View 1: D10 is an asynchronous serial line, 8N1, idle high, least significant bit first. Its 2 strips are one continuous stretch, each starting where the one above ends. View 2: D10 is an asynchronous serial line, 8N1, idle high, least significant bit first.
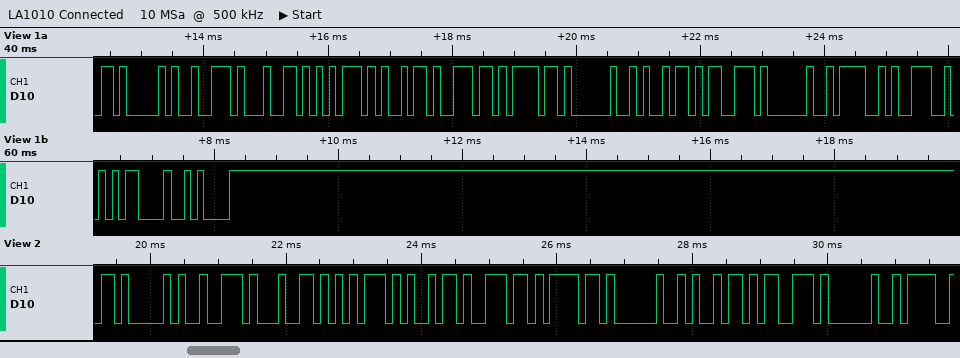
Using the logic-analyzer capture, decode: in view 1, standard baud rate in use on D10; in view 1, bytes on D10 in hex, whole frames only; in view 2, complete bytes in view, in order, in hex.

9600 baud
41 72 64 75 69 6E 6F 20 69 73 20 4F 4E 0D 0A
41 72 64 75 69 6E 6F 20 69 73 20
